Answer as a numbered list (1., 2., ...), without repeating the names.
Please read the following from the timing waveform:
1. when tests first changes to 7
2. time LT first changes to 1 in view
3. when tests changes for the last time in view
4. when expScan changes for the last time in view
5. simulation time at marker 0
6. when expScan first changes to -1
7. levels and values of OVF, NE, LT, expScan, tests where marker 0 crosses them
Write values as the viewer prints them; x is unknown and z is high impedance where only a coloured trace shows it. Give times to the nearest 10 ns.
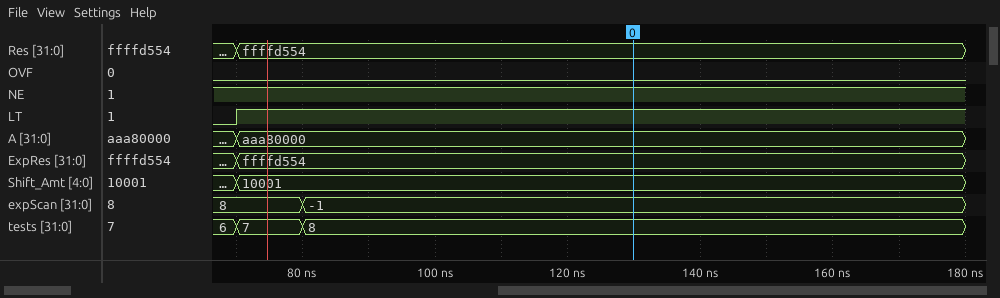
1. 70 ns
2. 70 ns
3. 80 ns
4. 80 ns
5. 130 ns
6. 80 ns
7. OVF=0, NE=1, LT=1, expScan=-1, tests=8
